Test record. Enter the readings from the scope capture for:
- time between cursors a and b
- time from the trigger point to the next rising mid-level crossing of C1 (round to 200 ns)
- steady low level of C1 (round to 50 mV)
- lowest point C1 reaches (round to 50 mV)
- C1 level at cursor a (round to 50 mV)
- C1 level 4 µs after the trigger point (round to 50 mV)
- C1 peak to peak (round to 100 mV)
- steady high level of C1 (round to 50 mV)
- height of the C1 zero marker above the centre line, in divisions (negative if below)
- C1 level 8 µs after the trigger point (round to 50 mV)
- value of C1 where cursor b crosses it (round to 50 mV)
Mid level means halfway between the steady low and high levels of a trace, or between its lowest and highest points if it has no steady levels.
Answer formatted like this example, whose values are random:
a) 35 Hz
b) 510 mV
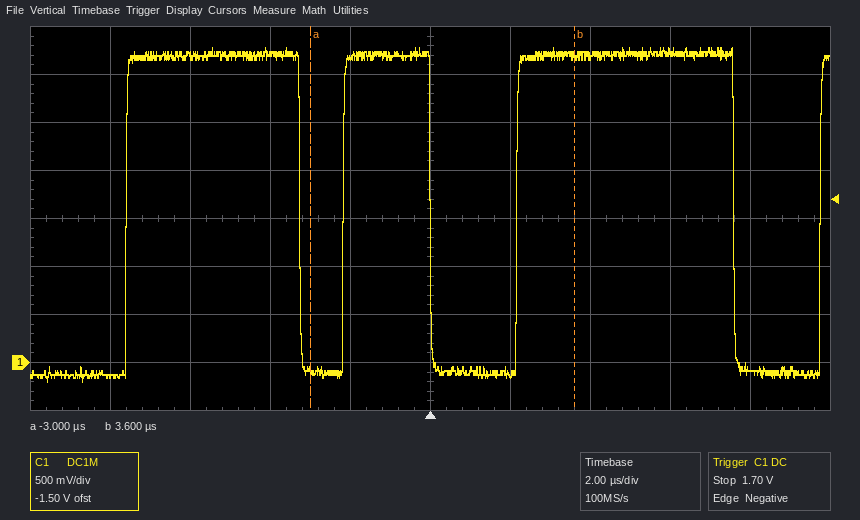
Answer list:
a) 6.6 µs
b) 2.2 µs
c) -100 mV
d) -200 mV
e) -100 mV
f) 3.20 V
g) 3.50 V
h) 3.20 V
i) -3.0 div
j) -100 mV
k) 3.20 V
